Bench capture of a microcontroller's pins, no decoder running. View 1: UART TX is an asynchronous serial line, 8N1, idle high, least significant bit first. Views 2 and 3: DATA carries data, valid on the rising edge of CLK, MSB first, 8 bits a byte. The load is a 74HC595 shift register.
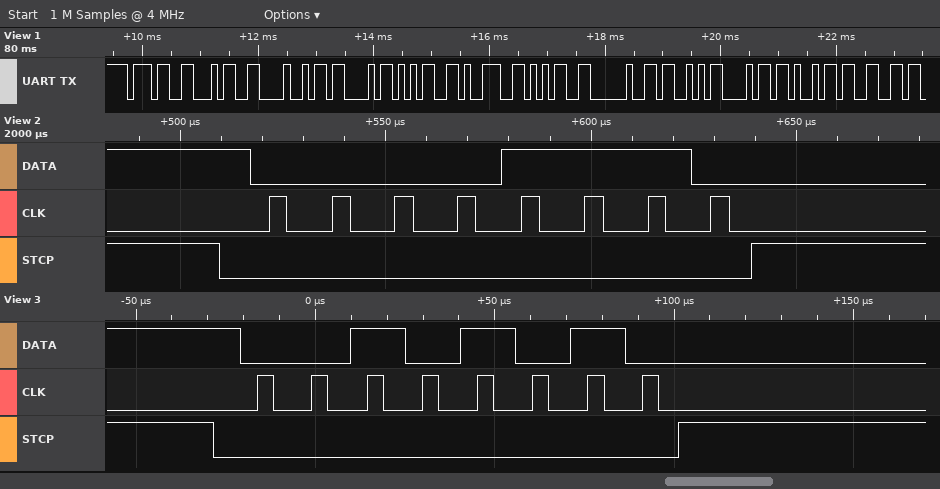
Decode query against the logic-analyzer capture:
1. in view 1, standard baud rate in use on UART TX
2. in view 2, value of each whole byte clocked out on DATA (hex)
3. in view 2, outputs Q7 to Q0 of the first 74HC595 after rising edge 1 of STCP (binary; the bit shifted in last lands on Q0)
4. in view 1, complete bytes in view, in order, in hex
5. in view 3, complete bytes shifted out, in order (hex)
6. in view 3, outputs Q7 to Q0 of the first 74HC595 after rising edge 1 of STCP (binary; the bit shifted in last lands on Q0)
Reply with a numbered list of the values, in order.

1. 9600 baud
2. 0E
3. 00001110
4. 0x37 0x34 0x48 0x43 0x35 0x39 0x35 0x20 0x53 0x68 0x69 0x66
5. 2A
6. 00101010
